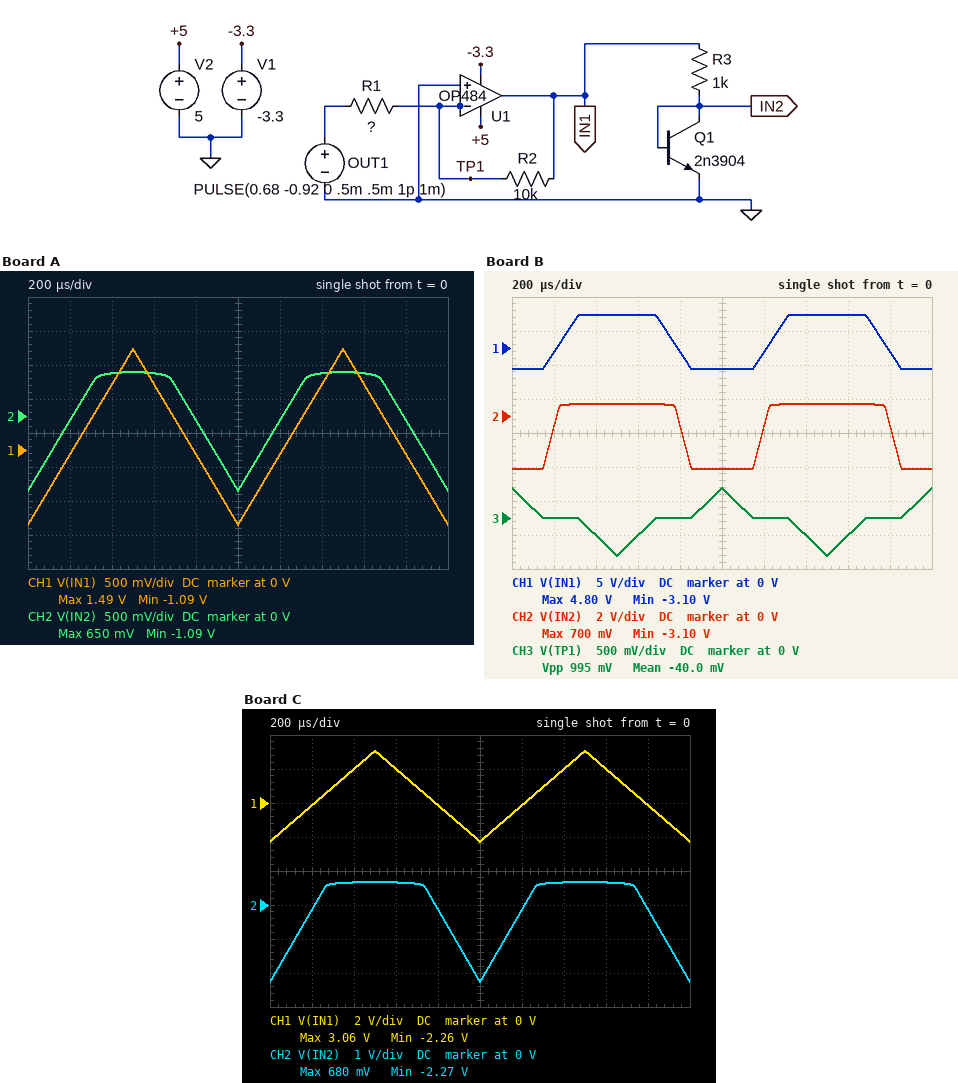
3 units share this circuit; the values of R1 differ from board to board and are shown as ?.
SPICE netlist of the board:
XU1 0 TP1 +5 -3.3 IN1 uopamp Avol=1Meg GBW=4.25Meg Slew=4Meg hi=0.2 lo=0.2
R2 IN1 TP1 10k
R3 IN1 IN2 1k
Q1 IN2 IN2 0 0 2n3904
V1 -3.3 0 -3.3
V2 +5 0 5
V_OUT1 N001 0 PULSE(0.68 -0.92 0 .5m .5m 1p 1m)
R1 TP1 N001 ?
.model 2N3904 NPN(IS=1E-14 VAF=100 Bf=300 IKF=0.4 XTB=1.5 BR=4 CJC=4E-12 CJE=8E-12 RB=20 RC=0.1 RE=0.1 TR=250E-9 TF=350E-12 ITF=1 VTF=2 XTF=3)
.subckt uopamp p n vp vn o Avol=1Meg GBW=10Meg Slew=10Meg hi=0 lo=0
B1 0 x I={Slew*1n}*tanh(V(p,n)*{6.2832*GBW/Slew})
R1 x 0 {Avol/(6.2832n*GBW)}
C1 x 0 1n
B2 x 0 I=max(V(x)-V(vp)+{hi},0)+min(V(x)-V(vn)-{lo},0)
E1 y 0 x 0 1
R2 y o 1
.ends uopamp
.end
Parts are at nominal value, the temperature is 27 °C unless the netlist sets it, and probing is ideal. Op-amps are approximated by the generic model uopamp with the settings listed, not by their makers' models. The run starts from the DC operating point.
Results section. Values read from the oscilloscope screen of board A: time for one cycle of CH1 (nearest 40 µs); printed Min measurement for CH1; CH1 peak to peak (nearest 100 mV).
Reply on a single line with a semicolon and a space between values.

1.00 ms; -1.09 V; 2.6 V
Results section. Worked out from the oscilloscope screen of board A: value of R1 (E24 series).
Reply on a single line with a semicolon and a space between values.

6.2 kΩ
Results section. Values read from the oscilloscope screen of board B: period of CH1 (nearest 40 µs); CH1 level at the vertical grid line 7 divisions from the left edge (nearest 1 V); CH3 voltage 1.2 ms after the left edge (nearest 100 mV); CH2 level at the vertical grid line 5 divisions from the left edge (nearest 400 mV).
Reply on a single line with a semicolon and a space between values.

1.00 ms; 5 V; 0 V; -3.2 V
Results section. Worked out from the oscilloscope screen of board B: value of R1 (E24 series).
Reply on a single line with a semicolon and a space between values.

680 Ω
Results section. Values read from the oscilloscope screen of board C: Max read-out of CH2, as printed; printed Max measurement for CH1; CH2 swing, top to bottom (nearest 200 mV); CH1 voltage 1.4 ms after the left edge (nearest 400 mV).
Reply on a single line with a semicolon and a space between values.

680 mV; 3.06 V; 3.0 V; 2.0 V
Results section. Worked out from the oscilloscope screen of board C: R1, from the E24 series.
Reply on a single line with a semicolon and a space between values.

3 kΩ
